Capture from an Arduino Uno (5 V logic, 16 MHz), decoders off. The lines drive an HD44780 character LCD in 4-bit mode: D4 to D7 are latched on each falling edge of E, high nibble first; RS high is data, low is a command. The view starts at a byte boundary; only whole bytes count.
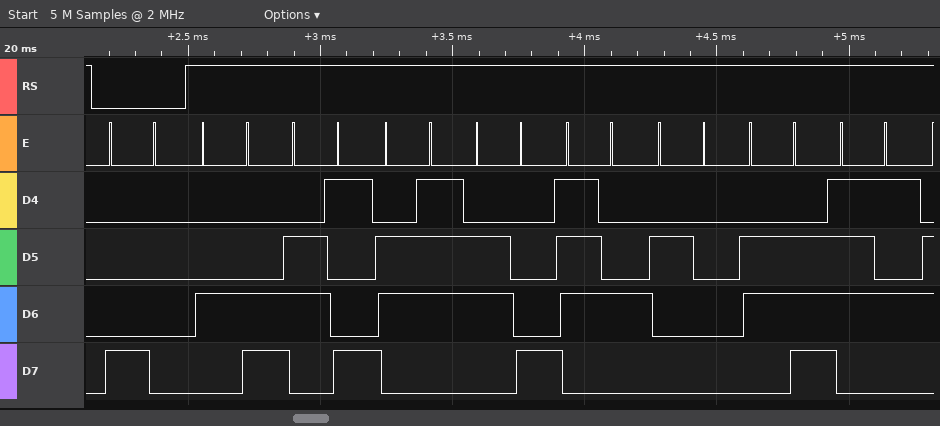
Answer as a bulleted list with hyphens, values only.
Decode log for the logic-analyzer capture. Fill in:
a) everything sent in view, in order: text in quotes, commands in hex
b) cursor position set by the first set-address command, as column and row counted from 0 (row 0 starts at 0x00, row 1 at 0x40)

- 0x80 "Light nu"
- column 0, row 0
